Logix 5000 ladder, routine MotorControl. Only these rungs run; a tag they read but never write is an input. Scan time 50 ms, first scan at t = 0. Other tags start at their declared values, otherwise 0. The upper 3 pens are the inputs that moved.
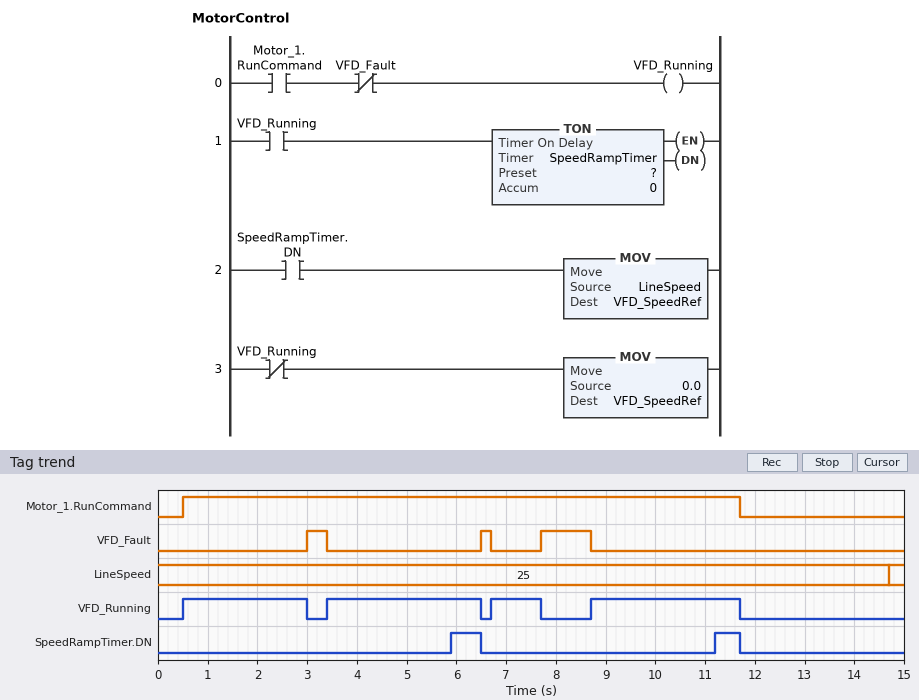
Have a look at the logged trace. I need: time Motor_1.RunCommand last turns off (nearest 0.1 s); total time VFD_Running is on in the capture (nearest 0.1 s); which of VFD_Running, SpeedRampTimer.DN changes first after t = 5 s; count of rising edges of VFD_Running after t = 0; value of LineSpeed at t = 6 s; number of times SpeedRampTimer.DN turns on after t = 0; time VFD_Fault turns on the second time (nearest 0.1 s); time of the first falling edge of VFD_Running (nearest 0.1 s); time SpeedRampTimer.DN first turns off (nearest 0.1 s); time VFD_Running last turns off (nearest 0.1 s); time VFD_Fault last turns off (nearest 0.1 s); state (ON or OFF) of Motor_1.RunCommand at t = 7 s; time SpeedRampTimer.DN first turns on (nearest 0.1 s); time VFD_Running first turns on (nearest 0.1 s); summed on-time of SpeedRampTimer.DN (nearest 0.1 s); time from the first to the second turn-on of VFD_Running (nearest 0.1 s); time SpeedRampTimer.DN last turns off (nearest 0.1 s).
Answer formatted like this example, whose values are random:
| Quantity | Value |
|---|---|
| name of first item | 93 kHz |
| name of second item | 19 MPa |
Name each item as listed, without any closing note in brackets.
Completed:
| Quantity | Value |
|---|---|
| time Motor_1.RunCommand last turns off | 11.7 s |
| total time VFD_Running is on in the capture | 9.6 s |
| which of VFD_Running, SpeedRampTimer.DN changes first after t = 5 s | SpeedRampTimer.DN |
| count of rising edges of VFD_Running after t = 0 | 4 |
| value of LineSpeed at t = 6 s | 25 |
| number of times SpeedRampTimer.DN turns on after t = 0 | 2 |
| time VFD_Fault turns on the second time | 6.5 s |
| time of the first falling edge of VFD_Running | 3.0 s |
| time SpeedRampTimer.DN first turns off | 6.5 s |
| time VFD_Running last turns off | 11.7 s |
| time VFD_Fault last turns off | 8.7 s |
| state (ON or OFF) of Motor_1.RunCommand at t = 7 s | ON |
| time SpeedRampTimer.DN first turns on | 5.9 s |
| time VFD_Running first turns on | 0.5 s |
| summed on-time of SpeedRampTimer.DN | 1.1 s |
| time from the first to the second turn-on of VFD_Running | 2.9 s |
| time SpeedRampTimer.DN last turns off | 11.7 s |
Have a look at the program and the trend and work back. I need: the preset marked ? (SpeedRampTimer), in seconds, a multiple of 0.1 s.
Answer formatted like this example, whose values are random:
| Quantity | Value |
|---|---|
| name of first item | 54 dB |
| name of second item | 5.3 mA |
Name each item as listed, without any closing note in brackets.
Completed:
| Quantity | Value |
|---|---|
| the preset marked ? (SpeedRampTimer), in seconds, a multiple of 0.1 s | 2.5 s |
